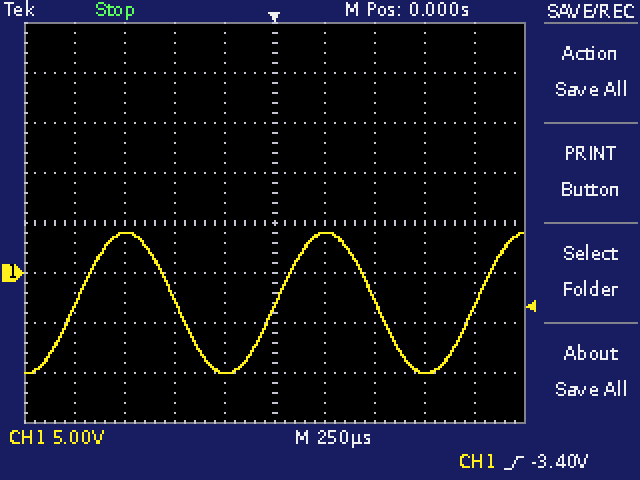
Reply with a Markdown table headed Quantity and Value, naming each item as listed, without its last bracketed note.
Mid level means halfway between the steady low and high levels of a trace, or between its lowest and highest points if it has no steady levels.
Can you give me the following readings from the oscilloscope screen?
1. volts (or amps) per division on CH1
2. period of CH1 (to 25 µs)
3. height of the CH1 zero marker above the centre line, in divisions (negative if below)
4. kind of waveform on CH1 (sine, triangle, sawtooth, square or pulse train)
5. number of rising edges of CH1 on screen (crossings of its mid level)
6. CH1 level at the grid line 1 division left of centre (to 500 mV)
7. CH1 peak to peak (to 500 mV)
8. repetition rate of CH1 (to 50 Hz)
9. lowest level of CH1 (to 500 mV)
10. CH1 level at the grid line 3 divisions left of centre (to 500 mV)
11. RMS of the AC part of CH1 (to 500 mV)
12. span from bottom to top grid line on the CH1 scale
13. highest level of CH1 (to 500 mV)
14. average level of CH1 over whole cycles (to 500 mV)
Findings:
| Quantity | Value |
|---|---|
| volts (or amps) per division on CH1 | 5 V |
| period of CH1 | 1.000 ms |
| height of the CH1 zero marker above the centre line, in divisions | -1.0 div |
| kind of waveform on CH1 | sine |
| number of rising edges of CH1 on screen | 3 |
| CH1 level at the grid line 1 division left of centre | -10.0 V |
| CH1 peak to peak | 14.0 V |
| repetition rate of CH1 | 1.00 kHz |
| lowest level of CH1 | -10.0 V |
| CH1 level at the grid line 3 divisions left of centre | 4.0 V |
| RMS of the AC part of CH1 | 5.0 V |
| span from bottom to top grid line on the CH1 scale | 40 V |
| highest level of CH1 | 4.0 V |
| average level of CH1 over whole cycles | -3.0 V |
